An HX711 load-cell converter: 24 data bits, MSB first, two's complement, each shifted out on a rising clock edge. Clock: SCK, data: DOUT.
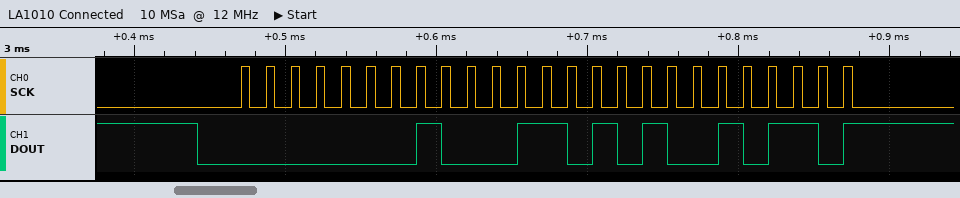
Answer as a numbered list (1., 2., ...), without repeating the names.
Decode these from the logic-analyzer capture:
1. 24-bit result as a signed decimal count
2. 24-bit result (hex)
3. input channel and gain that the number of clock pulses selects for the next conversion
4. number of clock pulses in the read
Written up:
1. 72342
2. 0x011A96
3. channel A, gain 128
4. 25
